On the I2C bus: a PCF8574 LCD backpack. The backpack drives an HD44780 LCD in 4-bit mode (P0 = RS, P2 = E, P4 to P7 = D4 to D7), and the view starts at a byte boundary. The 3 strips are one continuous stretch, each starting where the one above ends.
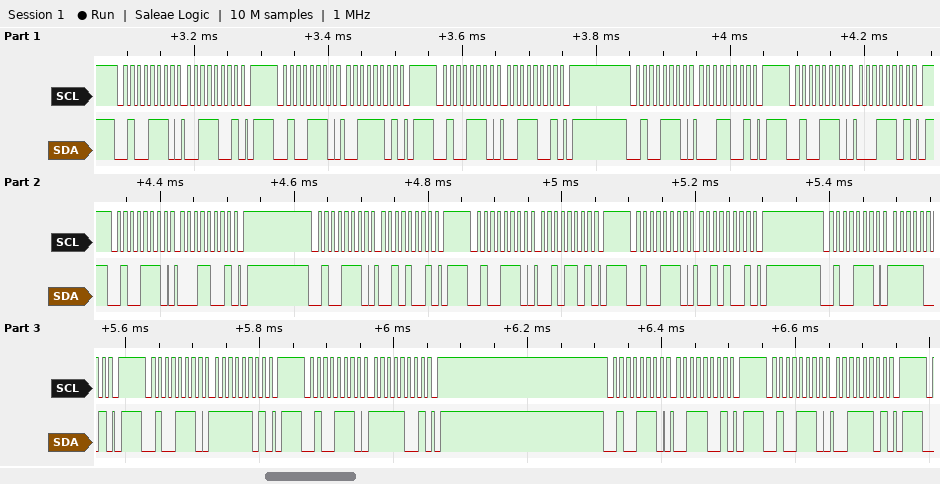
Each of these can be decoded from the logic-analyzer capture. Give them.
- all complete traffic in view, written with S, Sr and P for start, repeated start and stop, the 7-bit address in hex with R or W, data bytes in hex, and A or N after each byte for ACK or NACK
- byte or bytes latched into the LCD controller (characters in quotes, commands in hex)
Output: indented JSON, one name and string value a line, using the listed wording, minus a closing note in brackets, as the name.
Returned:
{
  "all complete traffic in view, written with S, Sr and P for start, repeated start and stop, the 7-bit address in hex with R or W, data bytes in hex, and A or N after each byte for ACK or NACK": "S 27W A 39 A P S 27W A 3D A P S 27W A 39 A P S 27W A 19 A P S 27W A 1D A P S 27W A 19 A P S 27W A 29 A P S 27W A 2D A P S 27W A 29 A P S 27W A F9 A P S 27W A FD A P S 27W A F9 A P S 27W A 39 A P S 27W A 3D A P",
  "byte or bytes latched into the LCD controller": "'1' '/'"
}
